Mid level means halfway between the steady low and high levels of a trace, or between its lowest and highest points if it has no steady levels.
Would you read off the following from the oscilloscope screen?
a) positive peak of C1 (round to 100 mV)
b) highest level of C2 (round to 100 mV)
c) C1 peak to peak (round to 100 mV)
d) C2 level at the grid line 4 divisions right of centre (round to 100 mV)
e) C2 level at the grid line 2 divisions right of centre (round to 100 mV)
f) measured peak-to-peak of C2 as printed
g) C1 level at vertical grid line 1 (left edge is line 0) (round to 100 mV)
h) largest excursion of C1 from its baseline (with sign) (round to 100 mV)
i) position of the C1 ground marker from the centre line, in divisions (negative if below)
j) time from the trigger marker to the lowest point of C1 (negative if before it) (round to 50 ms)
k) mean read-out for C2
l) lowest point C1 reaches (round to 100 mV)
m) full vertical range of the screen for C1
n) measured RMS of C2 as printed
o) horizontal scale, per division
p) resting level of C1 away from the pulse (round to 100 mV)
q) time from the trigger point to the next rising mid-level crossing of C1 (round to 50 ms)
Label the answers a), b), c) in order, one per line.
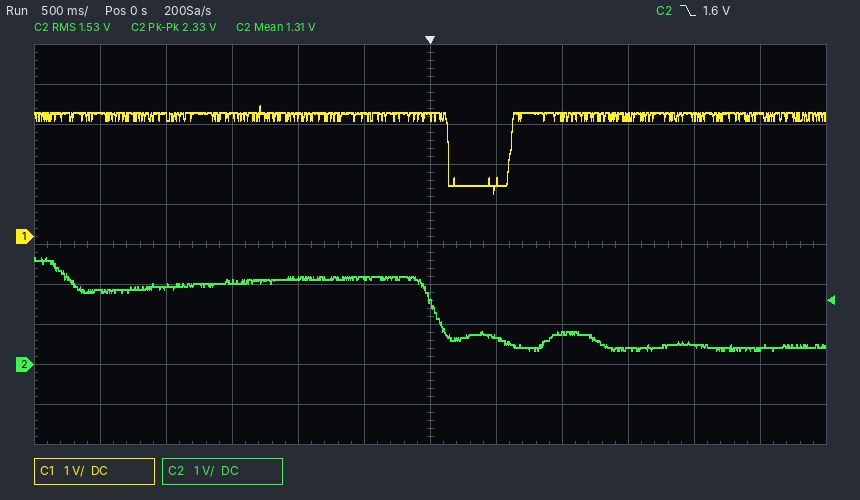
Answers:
a) 3.3 V
b) 2.7 V
c) 2.2 V
d) 500 mV
e) 800 mV
f) 2.33 V
g) 3.1 V
h) -2.0 V
i) +0.2 div
j) +500 ms
k) 1.31 V
l) 1.1 V
m) 10 V
n) 1.53 V
o) 500 ms
p) 3.1 V
q) 600 ms
